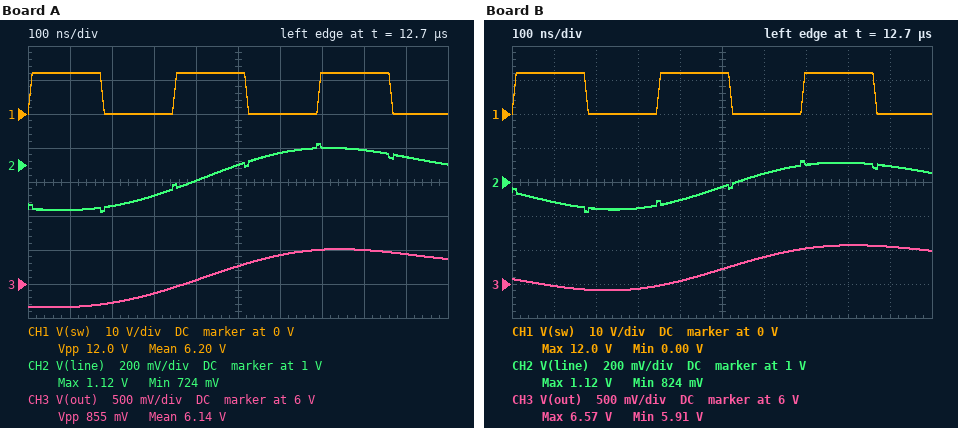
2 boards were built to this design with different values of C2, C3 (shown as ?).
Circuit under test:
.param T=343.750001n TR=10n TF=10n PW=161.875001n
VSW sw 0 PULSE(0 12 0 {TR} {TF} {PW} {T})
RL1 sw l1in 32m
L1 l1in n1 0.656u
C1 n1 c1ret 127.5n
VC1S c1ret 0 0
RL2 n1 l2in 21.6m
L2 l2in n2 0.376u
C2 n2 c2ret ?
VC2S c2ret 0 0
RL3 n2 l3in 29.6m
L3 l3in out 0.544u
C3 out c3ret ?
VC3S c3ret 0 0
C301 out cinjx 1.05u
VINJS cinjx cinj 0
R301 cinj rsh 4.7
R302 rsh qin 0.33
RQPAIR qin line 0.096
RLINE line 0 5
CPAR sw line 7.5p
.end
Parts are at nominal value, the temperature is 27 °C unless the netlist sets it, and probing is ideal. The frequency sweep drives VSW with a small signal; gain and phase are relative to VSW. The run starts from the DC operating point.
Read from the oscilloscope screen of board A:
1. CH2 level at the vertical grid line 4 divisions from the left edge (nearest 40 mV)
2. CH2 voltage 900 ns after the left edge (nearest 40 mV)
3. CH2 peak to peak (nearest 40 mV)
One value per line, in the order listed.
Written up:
920 mV
1.04 V
400 mV
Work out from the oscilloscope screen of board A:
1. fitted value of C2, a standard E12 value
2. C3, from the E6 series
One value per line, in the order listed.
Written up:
220 nF
100 nF
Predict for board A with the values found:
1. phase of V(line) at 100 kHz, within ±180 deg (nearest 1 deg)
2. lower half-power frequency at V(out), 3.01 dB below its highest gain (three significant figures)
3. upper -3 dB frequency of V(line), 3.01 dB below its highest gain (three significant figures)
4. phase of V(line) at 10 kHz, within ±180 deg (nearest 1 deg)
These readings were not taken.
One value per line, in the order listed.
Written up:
1 deg
218 kHz
278 kHz
56 deg
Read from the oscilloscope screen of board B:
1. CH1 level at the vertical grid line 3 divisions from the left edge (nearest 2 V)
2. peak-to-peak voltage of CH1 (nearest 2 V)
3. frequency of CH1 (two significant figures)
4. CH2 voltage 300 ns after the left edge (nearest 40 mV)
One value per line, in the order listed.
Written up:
0 V
12 V
2.9 MHz
840 mV
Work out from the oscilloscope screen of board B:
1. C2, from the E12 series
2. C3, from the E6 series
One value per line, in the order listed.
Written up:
120 nF
150 nF
